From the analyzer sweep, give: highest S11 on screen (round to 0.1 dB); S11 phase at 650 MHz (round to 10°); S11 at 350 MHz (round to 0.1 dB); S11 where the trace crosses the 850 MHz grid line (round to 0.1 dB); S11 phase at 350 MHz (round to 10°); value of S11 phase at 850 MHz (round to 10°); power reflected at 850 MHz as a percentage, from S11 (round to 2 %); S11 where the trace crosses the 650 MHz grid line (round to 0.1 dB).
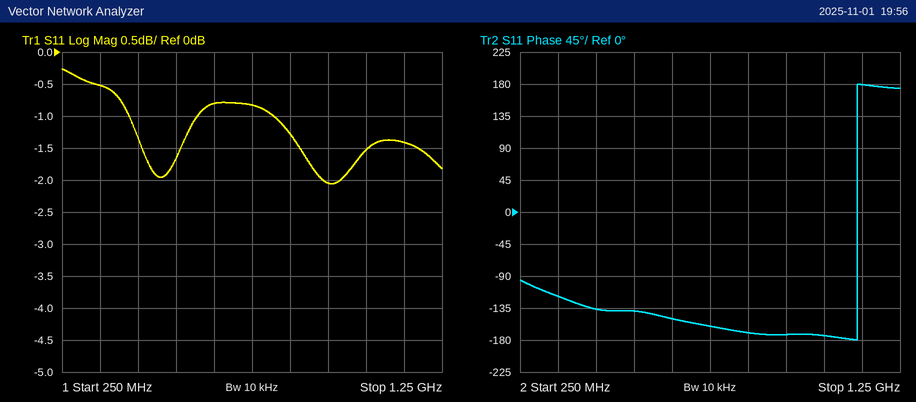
-0.3 dB
-150°
-0.5 dB
-1.3 dB
-120°
-170°
74 %
-0.8 dB
